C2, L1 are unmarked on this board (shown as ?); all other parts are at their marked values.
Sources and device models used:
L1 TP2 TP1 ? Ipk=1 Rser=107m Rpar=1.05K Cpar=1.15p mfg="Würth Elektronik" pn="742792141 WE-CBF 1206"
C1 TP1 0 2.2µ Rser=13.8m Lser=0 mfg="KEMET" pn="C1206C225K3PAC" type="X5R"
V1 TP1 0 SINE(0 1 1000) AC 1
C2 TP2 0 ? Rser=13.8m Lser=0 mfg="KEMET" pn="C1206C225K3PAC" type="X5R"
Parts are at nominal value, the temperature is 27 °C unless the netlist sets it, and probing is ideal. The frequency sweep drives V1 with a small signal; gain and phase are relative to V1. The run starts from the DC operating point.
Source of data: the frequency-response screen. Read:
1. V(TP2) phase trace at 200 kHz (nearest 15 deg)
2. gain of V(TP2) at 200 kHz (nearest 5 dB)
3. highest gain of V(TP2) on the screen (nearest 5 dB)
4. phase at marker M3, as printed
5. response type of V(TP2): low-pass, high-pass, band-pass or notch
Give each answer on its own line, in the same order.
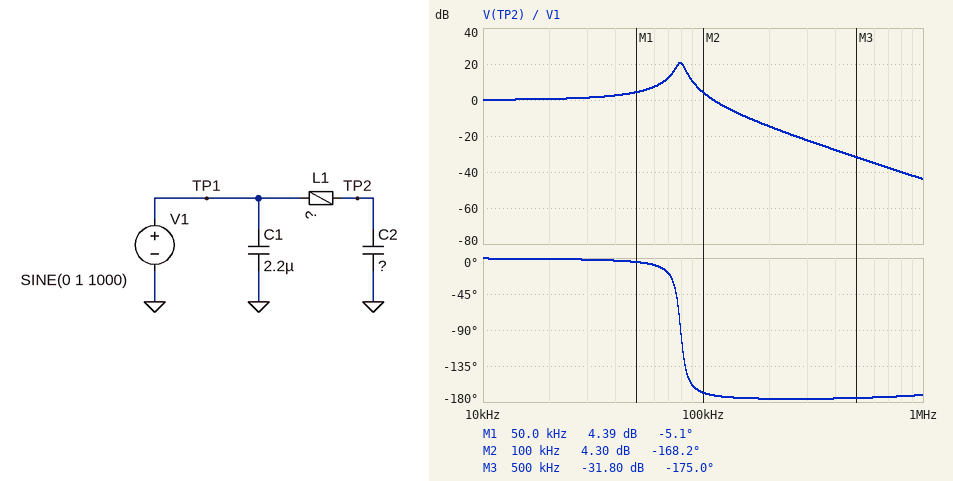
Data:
-180 deg
-15 dB
20 dB
-175.0 deg
low-pass
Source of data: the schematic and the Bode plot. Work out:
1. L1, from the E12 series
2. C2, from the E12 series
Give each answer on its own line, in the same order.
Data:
2.7 µH
1.5 µF
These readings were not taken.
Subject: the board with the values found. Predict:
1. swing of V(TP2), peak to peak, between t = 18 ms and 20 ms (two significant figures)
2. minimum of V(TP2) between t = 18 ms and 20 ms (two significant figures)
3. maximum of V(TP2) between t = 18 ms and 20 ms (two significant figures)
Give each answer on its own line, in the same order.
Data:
2.0 V
-1.0 V
1.0 V
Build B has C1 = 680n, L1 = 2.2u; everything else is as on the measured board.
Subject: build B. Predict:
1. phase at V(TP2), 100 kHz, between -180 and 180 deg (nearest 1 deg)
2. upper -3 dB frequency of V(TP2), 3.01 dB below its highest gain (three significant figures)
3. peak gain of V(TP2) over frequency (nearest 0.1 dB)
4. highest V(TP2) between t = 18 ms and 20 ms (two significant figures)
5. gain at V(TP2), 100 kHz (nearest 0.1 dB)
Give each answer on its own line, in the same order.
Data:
-158 deg
91.7 kHz
19.9 dB
1.0 V
9.8 dB
